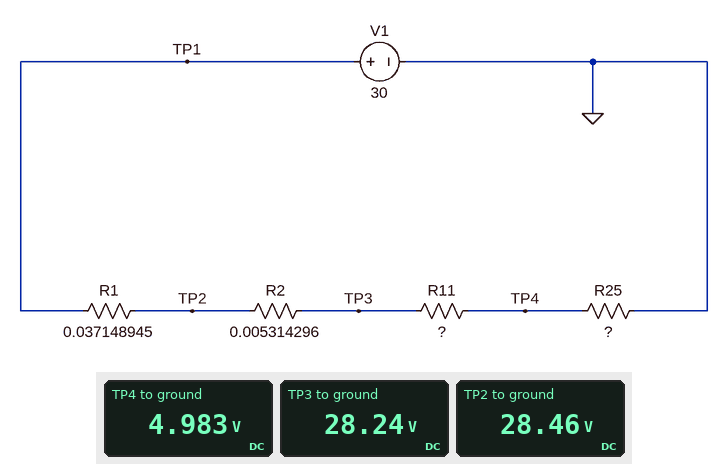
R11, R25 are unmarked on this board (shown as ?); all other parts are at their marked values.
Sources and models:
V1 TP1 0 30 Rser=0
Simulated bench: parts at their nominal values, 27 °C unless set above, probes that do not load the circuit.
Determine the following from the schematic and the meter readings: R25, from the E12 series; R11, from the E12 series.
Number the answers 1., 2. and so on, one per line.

1. 0.12 Ω
2. 0.56 Ω
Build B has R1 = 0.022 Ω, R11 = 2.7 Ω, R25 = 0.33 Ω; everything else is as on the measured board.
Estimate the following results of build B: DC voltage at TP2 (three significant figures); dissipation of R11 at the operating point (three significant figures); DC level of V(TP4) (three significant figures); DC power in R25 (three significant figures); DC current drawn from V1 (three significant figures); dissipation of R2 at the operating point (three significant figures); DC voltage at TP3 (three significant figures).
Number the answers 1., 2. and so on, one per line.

1. 29.8 V
2. 260 W
3. 3.24 V
4. 31.8 W
5. 9.81 A
6. 512 mW
7. 29.7 V
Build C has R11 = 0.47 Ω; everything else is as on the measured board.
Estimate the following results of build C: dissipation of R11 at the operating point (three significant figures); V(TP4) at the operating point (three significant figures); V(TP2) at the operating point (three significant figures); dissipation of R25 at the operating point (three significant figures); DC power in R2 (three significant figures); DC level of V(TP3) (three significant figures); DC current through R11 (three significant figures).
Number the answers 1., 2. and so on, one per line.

1. 1.06 kW
2. 5.69 V
3. 28.2 V
4. 270 W
5. 12.0 W
6. 28.0 V
7. 47.4 A
